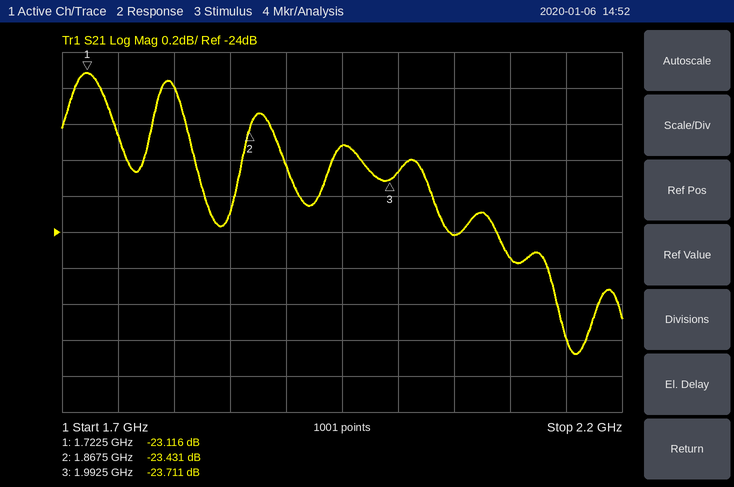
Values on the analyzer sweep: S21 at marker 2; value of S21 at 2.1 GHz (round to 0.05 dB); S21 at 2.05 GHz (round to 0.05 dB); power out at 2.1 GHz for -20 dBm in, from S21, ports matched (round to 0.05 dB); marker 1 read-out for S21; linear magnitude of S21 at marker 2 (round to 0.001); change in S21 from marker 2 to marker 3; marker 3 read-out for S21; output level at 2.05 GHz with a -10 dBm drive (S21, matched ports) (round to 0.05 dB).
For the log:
-23.431 dB
-24.15 dB
-24.00 dB
-44.15 dBm
-23.116 dB
0.067
-0.280 dB
-23.711 dB
-34.00 dBm
